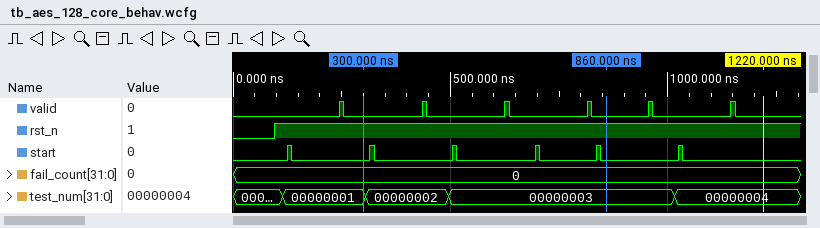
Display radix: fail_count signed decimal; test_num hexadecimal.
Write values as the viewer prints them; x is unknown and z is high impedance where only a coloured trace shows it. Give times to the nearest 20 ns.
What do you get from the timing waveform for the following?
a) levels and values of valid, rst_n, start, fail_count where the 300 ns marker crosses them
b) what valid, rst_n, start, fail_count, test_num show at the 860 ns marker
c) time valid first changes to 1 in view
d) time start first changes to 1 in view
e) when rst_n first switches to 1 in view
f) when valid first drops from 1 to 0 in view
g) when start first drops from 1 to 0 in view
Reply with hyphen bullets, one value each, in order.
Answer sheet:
- valid=0, rst_n=1, start=0, fail_count=0
- valid=0, rst_n=1, start=0, fail_count=0, test_num=00000003
- 240 ns
- 120 ns
- 100 ns
- 260 ns
- 140 ns
